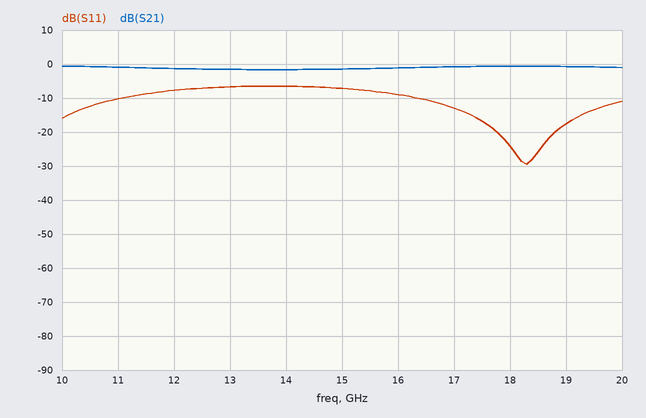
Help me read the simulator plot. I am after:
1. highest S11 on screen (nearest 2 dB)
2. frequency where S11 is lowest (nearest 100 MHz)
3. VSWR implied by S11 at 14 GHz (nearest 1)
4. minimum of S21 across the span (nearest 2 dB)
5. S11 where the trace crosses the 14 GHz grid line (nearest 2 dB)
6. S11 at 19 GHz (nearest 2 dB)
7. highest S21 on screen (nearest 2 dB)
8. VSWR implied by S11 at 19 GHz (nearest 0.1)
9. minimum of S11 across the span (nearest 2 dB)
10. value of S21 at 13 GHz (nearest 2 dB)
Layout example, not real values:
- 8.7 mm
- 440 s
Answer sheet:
- -6 dB
- 18.3 GHz
- 3
- -2 dB
- -6 dB
- -18 dB
- 0 dB
- 1.3
- -30 dB
- -2 dB
